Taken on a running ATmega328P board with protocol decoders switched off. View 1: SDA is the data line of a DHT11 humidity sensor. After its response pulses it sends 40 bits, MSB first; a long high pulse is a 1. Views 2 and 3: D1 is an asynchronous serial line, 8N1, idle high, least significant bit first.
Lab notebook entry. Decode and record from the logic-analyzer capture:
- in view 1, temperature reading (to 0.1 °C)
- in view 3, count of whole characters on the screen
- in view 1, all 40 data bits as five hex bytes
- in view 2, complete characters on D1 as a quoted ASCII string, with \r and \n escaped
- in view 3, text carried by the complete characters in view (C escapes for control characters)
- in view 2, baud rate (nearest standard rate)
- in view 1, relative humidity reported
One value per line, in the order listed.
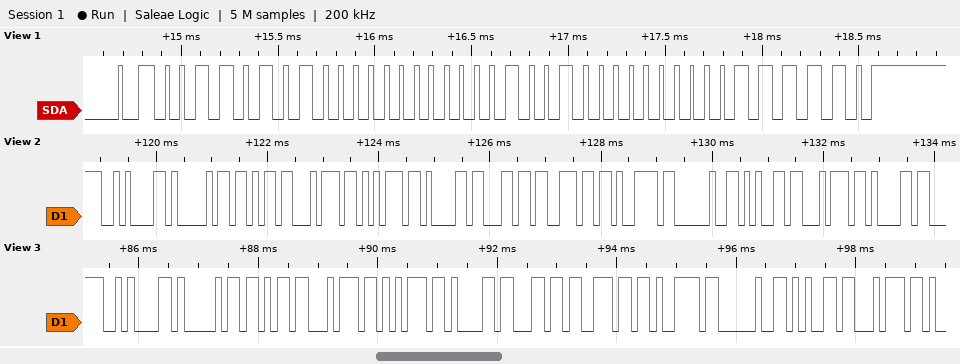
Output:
9.0 °C
12
35 00 09 00 3E
"\nAktualny eta"
"\nAktualny et"
9600 baud
53 %
